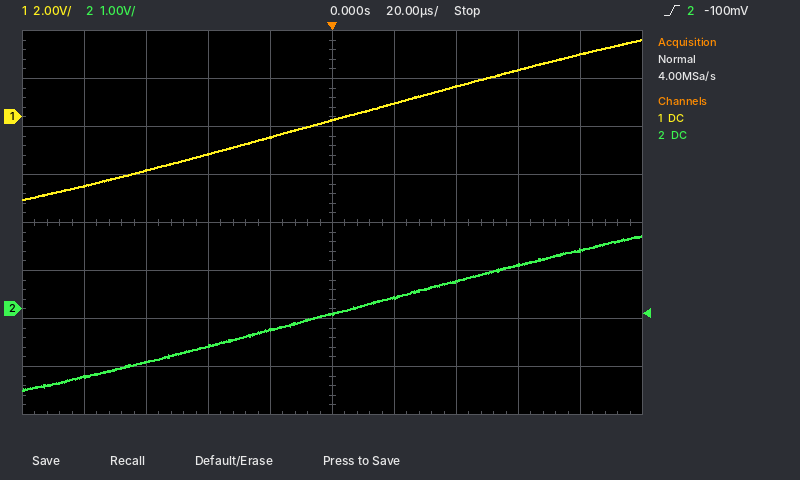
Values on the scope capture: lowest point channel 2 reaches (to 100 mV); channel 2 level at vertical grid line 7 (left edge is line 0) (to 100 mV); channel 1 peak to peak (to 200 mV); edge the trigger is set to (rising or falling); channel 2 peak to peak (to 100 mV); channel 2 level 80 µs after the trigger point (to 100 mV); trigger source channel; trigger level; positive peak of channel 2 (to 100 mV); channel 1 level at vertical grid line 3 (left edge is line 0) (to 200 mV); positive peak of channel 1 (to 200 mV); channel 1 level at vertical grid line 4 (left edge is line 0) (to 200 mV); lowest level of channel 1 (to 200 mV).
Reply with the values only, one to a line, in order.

-1.7 V
600 mV
6.6 V
rising
3.2 V
1.2 V
channel 2
-100 mV
1.5 V
-1.6 V
3.2 V
-800 mV
-3.4 V
